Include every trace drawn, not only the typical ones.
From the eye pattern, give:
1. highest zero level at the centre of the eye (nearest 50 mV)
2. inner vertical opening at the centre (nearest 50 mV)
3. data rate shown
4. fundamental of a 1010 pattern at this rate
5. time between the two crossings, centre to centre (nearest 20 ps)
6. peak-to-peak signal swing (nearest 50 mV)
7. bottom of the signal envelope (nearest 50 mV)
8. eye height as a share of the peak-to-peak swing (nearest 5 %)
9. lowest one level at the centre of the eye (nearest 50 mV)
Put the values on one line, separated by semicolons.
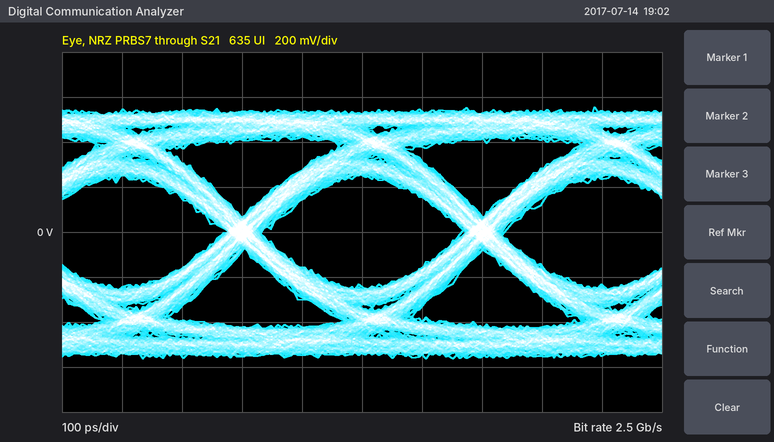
-250 mV; 500 mV; 2.5 Gb/s; 1.25 GHz; 400 ps; 1.10 V; -550 mV; 45 %; 250 mV
